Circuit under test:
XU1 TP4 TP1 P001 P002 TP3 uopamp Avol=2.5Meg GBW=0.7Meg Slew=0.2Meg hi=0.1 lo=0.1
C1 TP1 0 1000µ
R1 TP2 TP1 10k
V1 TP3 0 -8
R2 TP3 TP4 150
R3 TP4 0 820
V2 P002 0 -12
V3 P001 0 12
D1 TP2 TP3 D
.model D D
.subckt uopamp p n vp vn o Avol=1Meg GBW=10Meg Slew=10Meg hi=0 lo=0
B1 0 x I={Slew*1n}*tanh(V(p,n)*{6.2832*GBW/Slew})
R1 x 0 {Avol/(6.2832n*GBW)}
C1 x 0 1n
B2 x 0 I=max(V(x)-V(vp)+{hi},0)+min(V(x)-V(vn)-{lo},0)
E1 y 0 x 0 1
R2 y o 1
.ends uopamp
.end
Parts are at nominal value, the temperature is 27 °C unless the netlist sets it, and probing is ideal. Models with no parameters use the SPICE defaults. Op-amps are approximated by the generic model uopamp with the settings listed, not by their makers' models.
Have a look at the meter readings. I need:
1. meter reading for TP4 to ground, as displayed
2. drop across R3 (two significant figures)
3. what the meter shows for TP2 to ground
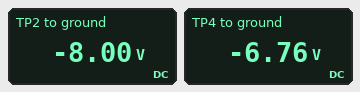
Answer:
-6.76 V
6.8 V
-8.00 V
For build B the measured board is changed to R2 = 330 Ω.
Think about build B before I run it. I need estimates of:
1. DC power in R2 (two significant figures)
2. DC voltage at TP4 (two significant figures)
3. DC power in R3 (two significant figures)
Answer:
16 mW
-5.7 V
40 mW
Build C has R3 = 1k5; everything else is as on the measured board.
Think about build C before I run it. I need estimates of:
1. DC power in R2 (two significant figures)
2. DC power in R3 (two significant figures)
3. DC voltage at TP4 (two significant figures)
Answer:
3.5 mW
35 mW
-7.3 V
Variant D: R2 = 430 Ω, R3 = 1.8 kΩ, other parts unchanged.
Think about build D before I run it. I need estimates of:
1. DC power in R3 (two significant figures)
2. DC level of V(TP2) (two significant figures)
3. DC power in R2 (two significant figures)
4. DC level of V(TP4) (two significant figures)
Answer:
23 mW
-8.0 V
5.5 mW
-6.5 V
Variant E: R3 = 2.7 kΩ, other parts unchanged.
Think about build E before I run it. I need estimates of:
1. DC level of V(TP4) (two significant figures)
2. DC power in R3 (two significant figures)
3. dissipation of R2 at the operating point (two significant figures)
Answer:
-7.6 V
21 mW
1.2 mW
